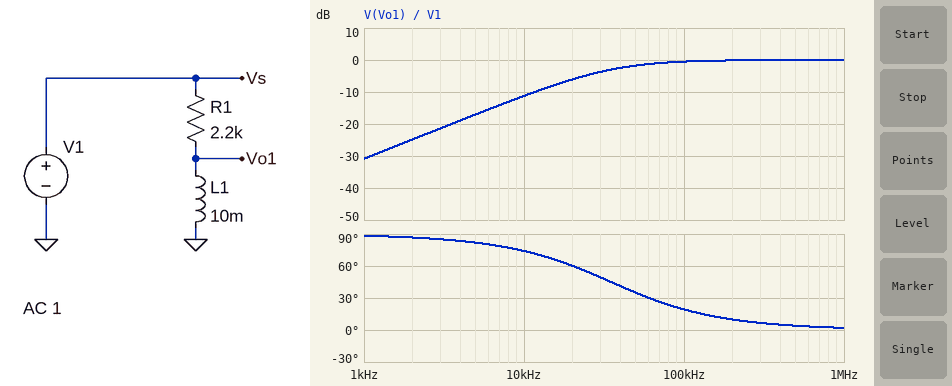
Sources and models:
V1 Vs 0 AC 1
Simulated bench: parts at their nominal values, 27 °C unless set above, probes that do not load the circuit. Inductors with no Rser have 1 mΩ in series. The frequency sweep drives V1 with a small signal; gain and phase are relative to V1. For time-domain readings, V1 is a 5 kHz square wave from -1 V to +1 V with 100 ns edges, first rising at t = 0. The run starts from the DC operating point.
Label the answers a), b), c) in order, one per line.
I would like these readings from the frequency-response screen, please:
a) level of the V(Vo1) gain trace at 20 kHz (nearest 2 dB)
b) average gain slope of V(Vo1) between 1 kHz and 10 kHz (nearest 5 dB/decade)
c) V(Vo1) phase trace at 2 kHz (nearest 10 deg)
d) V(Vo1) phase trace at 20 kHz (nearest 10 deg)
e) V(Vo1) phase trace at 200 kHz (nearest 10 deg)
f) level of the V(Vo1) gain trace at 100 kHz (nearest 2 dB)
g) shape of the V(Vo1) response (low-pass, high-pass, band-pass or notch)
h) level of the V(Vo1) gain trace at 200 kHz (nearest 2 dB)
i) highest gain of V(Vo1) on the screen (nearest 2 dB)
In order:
a) -6 dB
b) 20 dB/decade
c) 90 deg
d) 60 deg
e) 10 deg
f) 0 dB
g) high-pass
h) 0 dB
i) 0 dB
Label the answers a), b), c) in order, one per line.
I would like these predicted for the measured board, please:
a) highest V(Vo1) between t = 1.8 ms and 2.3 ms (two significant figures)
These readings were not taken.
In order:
a) 2.0 V
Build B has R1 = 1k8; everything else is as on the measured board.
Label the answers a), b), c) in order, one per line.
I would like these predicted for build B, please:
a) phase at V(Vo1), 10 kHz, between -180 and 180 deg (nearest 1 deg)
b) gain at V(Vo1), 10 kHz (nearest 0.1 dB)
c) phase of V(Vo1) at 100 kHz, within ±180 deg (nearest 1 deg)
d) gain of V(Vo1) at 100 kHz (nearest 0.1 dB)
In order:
a) 71 deg
b) -9.6 dB
c) 16 deg
d) -0.3 dB
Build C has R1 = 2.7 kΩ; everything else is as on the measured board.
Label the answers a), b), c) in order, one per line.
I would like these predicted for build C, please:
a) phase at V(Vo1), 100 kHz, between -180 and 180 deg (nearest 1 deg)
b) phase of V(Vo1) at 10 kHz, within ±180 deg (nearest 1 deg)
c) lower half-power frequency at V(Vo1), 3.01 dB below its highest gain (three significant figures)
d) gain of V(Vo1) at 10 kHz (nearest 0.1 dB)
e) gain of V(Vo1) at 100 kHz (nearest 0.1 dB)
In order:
a) 23 deg
b) 77 deg
c) 43.0 kHz
d) -12.9 dB
e) -0.7 dB
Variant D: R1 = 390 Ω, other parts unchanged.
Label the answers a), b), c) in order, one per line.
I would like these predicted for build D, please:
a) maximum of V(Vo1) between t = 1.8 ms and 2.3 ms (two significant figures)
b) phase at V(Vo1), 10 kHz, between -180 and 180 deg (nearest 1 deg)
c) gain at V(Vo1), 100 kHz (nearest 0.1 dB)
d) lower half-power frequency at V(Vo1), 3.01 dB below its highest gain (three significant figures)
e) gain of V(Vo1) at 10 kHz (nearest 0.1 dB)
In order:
a) 2.0 V
b) 32 deg
c) 0 dB
d) 6.21 kHz
e) -1.4 dB
